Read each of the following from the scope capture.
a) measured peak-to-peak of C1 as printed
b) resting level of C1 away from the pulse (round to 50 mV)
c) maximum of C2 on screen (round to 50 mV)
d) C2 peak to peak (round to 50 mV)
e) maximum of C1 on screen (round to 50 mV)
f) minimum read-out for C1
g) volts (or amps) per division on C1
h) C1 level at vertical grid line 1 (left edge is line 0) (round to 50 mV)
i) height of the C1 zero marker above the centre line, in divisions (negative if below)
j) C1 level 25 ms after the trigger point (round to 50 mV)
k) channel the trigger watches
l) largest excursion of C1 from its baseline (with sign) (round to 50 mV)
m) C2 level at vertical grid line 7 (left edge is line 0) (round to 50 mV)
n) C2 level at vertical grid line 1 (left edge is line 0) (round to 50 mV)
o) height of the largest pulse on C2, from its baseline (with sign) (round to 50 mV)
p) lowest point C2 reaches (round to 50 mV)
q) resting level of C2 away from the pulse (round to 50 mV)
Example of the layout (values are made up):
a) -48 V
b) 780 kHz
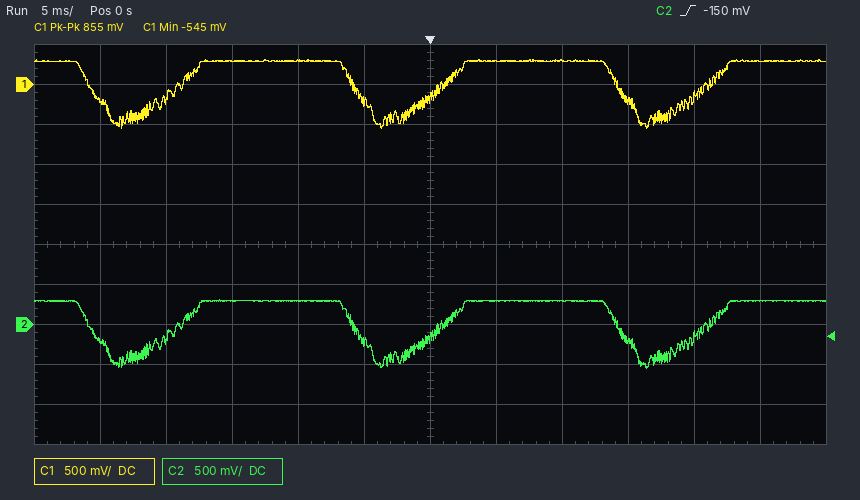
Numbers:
a) 855 mV
b) 300 mV
c) 300 mV
d) 850 mV
e) 300 mV
f) -545 mV
g) 500 mV
h) -200 mV
i) +4.0 div
j) 300 mV
k) C2
l) -850 mV
m) 300 mV
n) -200 mV
o) -850 mV
p) -550 mV
q) 300 mV
